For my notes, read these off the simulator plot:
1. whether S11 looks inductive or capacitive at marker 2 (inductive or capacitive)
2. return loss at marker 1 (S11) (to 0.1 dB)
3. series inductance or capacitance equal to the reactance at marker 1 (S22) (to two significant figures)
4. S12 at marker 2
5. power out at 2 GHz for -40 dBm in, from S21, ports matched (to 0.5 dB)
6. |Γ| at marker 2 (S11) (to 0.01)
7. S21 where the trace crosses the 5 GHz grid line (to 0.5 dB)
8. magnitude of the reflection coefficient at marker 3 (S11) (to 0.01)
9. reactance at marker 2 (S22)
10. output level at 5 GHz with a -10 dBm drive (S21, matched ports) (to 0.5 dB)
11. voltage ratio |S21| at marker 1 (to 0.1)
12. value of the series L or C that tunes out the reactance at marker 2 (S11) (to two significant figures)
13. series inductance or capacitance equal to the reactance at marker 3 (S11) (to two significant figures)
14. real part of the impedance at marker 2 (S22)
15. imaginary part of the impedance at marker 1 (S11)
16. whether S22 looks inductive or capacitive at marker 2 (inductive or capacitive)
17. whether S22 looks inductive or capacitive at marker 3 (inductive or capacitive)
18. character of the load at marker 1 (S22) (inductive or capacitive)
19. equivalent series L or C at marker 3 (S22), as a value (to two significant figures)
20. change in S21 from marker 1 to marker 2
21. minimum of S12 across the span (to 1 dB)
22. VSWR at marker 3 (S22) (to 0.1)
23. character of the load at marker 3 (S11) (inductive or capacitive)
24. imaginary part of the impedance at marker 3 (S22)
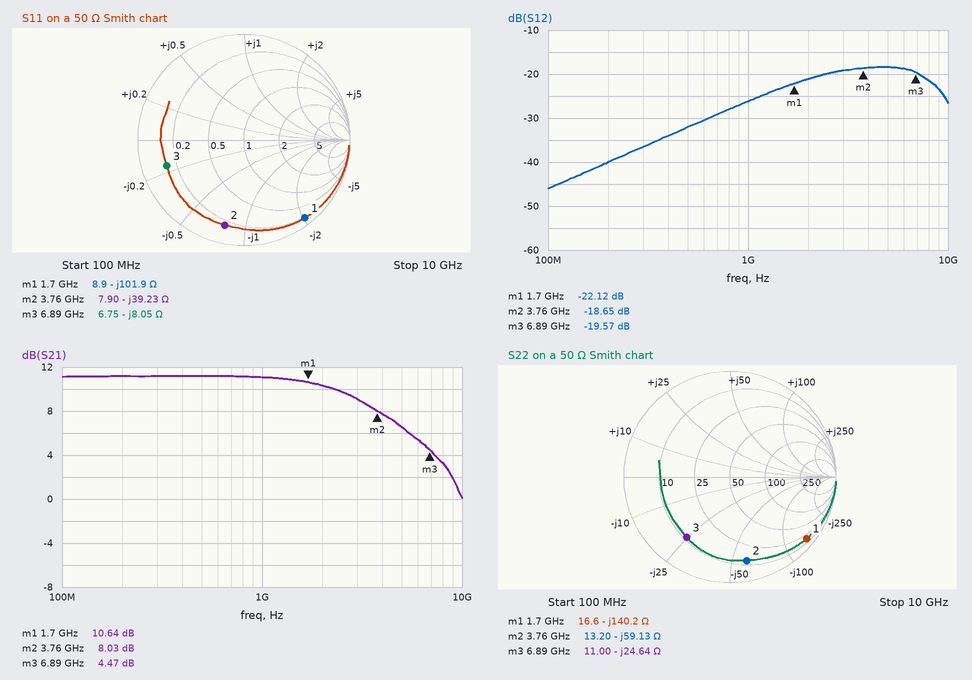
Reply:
capacitive
0.6 dB
670 fF
-18.65 dB
-29.5 dBm
0.82
6.5 dB
0.77
-59.13 Ω
-3.5 dBm
3.4
1.7 nH
2.9 pF
13.20 Ω
-101.9 Ω
capacitive
capacitive
capacitive
940 fF
-2.61 dB
-46 dB
5.7
capacitive
-24.64 Ω
